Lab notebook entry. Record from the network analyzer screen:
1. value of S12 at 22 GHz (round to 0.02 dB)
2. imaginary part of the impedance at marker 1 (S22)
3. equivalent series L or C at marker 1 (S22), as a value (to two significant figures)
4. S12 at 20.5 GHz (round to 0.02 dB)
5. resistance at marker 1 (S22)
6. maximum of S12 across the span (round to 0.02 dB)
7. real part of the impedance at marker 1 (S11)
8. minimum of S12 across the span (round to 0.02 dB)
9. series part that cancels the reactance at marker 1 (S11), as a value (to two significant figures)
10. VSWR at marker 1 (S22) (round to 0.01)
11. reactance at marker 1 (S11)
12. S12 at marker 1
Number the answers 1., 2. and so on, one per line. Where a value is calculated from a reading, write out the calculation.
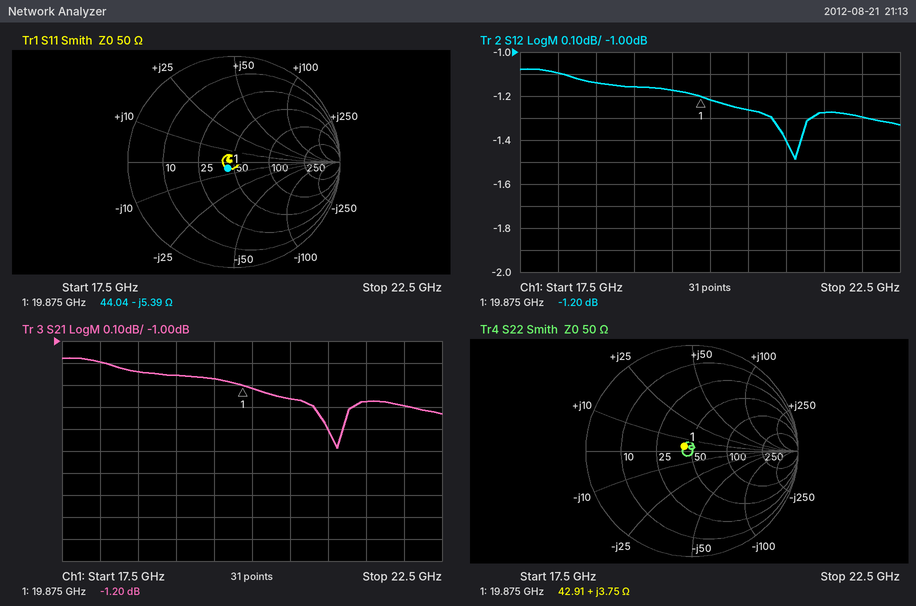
1. -1.30 dB
2. +3.75 Ω
3. L = 3.75 Ω/(2π × 19.875 GHz) ≈ 30 pH
4. -1.26 dB
5. 42.91 Ω
6. -1.08 dB
7. 44.04 Ω
8. -1.48 dB
9. L = 5.39 Ω/(2π × 19.875 GHz) ≈ 43 pH
10. 1.19
11. -5.39 Ω
12. -1.20 dB
